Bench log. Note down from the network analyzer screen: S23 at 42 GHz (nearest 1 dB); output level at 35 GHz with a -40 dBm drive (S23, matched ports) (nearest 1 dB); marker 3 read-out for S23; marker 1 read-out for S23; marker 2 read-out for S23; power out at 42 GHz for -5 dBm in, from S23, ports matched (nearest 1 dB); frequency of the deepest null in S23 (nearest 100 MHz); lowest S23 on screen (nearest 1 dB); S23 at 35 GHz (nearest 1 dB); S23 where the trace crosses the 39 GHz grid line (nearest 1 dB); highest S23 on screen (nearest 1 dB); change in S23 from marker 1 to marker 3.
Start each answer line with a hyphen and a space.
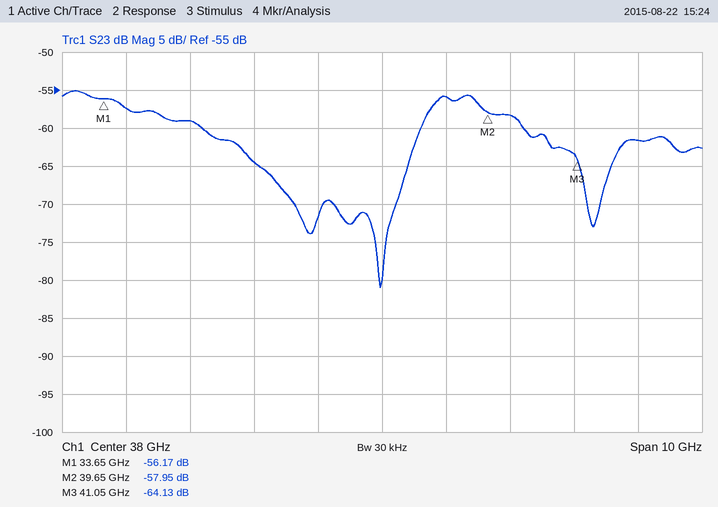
- -62 dB
- -99 dBm
- -64.13 dB
- -56.17 dB
- -57.95 dB
- -67 dBm
- 38.0 GHz
- -81 dB
- -59 dB
- -56 dB
- -55 dB
- -7.96 dB
